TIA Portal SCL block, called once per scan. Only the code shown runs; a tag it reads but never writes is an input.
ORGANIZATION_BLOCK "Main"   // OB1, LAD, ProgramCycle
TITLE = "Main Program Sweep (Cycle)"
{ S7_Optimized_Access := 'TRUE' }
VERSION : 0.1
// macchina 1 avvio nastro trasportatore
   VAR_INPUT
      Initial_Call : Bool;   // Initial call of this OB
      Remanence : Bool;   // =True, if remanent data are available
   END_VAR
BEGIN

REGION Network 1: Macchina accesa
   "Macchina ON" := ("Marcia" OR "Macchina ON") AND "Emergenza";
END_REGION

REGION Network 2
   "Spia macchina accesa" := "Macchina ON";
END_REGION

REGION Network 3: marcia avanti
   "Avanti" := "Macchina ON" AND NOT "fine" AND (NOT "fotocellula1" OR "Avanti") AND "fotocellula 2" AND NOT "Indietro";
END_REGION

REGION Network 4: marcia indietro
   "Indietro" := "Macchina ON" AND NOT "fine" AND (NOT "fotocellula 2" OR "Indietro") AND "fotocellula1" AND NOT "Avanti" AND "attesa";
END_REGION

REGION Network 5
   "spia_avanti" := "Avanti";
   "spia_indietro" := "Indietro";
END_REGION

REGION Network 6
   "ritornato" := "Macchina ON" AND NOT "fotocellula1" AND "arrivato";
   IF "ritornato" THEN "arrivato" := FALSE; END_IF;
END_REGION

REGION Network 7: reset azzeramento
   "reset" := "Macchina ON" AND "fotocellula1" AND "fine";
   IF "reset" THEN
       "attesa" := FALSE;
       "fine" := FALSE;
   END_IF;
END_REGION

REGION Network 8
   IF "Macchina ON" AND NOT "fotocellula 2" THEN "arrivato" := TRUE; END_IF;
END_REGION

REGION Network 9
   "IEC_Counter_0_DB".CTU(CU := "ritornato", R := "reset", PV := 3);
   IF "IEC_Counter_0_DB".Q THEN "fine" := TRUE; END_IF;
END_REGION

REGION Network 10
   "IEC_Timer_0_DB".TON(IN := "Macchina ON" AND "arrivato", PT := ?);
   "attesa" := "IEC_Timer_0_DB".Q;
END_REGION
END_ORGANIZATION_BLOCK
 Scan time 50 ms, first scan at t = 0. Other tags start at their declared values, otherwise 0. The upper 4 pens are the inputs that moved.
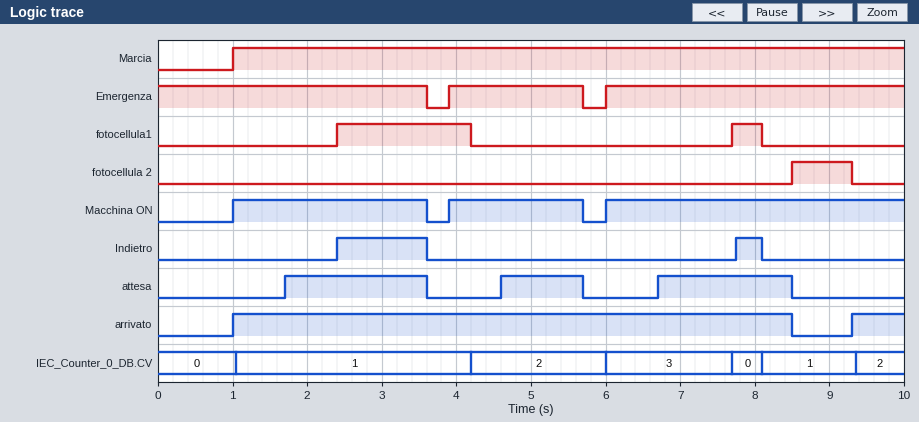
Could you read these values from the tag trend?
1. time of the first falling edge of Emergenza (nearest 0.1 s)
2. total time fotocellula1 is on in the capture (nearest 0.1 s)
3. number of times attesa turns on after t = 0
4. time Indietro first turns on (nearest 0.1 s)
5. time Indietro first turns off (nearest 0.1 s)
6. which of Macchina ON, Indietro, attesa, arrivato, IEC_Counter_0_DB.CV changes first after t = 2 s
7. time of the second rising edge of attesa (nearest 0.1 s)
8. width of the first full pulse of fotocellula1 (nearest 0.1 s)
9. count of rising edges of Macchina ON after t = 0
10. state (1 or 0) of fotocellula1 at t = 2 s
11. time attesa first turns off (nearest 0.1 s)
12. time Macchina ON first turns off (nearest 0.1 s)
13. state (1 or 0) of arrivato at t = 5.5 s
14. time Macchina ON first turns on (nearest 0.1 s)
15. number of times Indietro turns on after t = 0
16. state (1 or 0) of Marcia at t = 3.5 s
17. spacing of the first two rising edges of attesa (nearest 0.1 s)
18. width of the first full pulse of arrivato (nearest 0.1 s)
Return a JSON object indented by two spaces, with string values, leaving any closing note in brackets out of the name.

{
  "time of the first falling edge of Emergenza": "3.6 s",
  "total time fotocellula1 is on in the capture": "2.2 s",
  "number of times attesa turns on after t = 0": "3",
  "time Indietro first turns on": "2.4 s",
  "time Indietro first turns off": "3.6 s",
  "which of Macchina ON, Indietro, attesa, arrivato, IEC_Counter_0_DB.CV changes first after t = 2 s": "Indietro",
  "time of the second rising edge of attesa": "4.6 s",
  "width of the first full pulse of fotocellula1": "1.8 s",
  "count of rising edges of Macchina ON after t = 0": "3",
  "state (1 or 0) of fotocellula1 at t = 2 s": "0",
  "time attesa first turns off": "3.6 s",
  "time Macchina ON first turns off": "3.6 s",
  "state (1 or 0) of arrivato at t = 5.5 s": "1",
  "time Macchina ON first turns on": "1.0 s",
  "number of times Indietro turns on after t = 0": "2",
  "state (1 or 0) of Marcia at t = 3.5 s": "1",
  "spacing of the first two rising edges of attesa": "2.9 s",
  "width of the first full pulse of arrivato": "7.5 s"
}
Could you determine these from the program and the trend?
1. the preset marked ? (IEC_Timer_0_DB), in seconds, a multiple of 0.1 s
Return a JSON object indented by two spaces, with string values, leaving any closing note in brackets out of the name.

{
  "the preset marked ? (IEC_Timer_0_DB), in seconds, a multiple of 0.1 s": "0.7 s"
}
